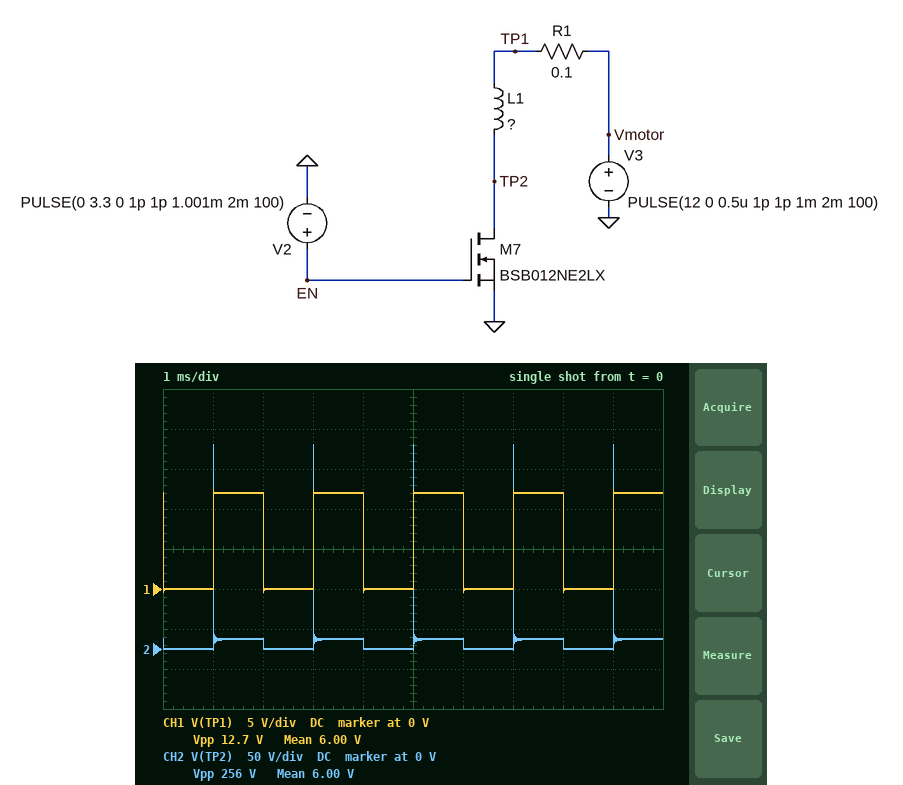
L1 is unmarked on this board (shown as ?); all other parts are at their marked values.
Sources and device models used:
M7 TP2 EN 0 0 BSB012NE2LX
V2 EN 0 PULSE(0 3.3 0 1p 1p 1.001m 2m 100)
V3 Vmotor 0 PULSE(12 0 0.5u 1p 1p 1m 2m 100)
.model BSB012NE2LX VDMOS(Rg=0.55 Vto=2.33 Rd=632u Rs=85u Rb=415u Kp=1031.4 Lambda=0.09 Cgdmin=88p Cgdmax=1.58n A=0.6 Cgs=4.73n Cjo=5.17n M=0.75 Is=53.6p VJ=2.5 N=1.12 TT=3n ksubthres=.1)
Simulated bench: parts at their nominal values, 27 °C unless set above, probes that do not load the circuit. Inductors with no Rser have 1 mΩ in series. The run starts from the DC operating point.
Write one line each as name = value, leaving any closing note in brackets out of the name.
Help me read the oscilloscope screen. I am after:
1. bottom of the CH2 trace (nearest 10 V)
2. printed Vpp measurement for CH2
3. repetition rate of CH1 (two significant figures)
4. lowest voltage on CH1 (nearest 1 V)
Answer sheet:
bottom of the CH2 trace = 0 V
printed Vpp measurement for CH2 = 256 V
repetition rate of CH1 = 500 Hz
lowest voltage on CH1 = 0 V
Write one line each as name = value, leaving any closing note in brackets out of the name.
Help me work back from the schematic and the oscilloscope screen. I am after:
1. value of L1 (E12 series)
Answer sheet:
value of L1 = 1.8 µH
